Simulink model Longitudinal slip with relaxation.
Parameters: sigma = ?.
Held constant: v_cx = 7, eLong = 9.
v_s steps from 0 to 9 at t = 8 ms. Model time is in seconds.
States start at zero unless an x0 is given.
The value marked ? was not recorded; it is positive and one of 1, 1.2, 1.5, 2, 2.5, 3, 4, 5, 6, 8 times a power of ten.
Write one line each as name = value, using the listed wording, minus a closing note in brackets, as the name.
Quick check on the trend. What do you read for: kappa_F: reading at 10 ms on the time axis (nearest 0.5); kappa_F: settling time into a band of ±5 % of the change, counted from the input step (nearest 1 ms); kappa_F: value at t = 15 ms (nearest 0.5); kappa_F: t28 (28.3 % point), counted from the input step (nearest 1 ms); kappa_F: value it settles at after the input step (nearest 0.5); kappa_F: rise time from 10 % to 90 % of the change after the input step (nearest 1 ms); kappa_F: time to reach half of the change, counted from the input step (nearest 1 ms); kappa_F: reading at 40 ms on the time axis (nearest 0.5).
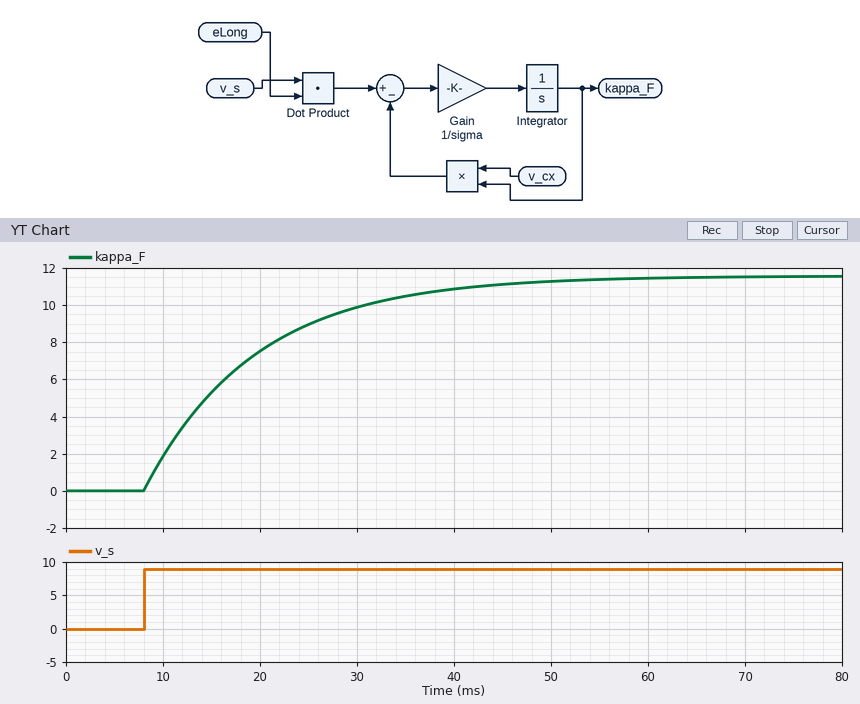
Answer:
kappa_F: reading at 10 ms on the time axis = 2.0
kappa_F: settling time into a band of ±5 % of the change, counted from the input step = 34 ms
kappa_F: value at t = 15 ms = 5.5
kappa_F: t28 (28.3 % point), counted from the input step = 4 ms
kappa_F: value it settles at after the input step = 11.5
kappa_F: rise time from 10 % to 90 % of the change after the input step = 25 ms
kappa_F: time to reach half of the change, counted from the input step = 8 ms
kappa_F: reading at 40 ms on the time axis = 11.0
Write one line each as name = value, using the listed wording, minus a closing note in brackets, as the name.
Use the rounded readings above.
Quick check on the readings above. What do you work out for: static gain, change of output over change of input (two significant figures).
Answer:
static gain, change of output over change of input = 1.3
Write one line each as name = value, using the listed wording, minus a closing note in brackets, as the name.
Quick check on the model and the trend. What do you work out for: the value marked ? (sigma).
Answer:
the value marked ? = 0.08
